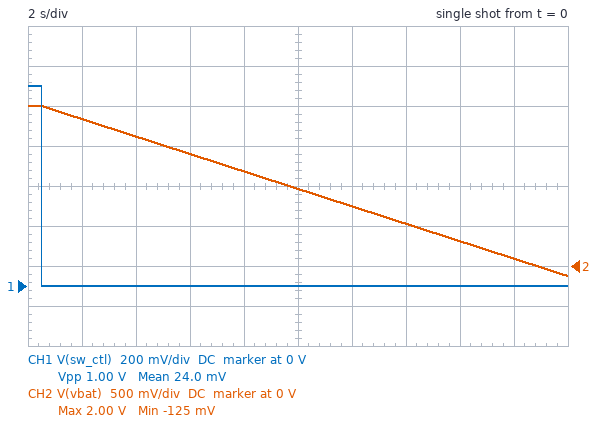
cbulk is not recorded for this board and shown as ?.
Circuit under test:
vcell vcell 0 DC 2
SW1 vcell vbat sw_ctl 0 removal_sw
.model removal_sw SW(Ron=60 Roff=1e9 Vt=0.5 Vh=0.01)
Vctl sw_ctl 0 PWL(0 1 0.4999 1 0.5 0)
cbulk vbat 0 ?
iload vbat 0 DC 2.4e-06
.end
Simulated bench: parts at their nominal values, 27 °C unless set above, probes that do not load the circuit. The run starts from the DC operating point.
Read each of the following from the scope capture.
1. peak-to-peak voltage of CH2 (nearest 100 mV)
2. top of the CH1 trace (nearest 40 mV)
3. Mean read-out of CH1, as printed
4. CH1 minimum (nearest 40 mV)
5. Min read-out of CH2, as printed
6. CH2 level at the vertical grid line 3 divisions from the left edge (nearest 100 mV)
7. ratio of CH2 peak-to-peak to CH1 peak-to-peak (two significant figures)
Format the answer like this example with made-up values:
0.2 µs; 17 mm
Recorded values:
2.1 V; 1.00 V; 24.0 mV; 0 V; -125 mV; 1.4 V; 2.1
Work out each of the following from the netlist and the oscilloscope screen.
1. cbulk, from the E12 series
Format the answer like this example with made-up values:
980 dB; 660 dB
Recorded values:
22 µF
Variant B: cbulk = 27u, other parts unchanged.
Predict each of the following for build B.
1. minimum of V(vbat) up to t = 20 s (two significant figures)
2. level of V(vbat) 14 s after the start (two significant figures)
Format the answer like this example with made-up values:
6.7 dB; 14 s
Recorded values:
270 mV; 800 mV
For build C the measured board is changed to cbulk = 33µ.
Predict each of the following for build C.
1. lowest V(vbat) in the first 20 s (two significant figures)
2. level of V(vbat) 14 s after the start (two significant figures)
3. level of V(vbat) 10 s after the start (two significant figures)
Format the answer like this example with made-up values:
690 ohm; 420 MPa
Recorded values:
580 mV; 1.0 V; 1.3 V
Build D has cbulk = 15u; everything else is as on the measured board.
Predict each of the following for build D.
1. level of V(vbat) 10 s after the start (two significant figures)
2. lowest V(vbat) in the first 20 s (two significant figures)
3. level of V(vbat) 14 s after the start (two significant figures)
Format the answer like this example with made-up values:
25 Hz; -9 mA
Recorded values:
480 mV; -1.1 V; -160 mV
